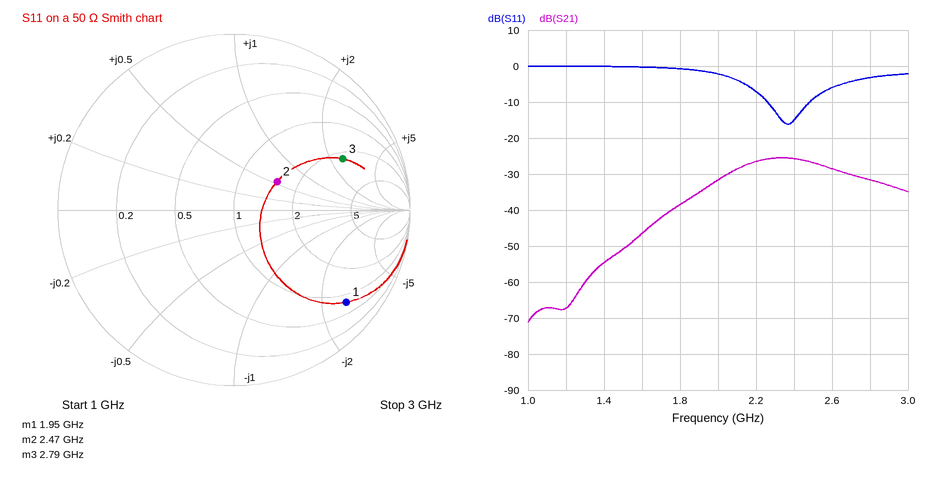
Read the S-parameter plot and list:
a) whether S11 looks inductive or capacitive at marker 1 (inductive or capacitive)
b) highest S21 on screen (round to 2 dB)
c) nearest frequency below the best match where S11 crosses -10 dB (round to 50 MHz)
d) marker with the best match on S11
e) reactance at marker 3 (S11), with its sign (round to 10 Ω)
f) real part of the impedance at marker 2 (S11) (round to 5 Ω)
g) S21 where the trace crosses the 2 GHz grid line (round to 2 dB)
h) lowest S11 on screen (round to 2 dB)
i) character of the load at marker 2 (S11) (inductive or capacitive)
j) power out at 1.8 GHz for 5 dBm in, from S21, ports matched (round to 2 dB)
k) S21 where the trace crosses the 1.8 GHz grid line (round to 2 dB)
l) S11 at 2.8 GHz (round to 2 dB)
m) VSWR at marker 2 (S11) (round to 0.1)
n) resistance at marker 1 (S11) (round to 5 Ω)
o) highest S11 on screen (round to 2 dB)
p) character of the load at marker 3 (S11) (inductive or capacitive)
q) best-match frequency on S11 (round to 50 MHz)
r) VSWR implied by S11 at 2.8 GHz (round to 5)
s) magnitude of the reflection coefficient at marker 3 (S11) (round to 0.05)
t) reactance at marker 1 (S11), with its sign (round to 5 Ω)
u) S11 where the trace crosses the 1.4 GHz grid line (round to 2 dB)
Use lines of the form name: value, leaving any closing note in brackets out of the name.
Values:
whether S11 looks inductive or capacitive at marker 1: capacitive
highest S21 on screen: -26 dB
nearest frequency below the best match where S11 crosses -10 dB: 2.25 GHz
marker with the best match on S11: marker 2
reactance at marker 3 (S11), with its sign: +130 Ω
real part of the impedance at marker 2 (S11): 75 Ω
S21 where the trace crosses the 2 GHz grid line: -32 dB
lowest S11 on screen: -16 dB
character of the load at marker 2 (S11): inductive
power out at 1.8 GHz for 5 dBm in, from S21, ports matched: -34 dBm
S21 where the trace crosses the 1.8 GHz grid line: -38 dB
S11 at 2.8 GHz: -4 dB
VSWR at marker 2 (S11): 1.8
resistance at marker 1 (S11): 40 Ω
highest S11 on screen: 0 dB
character of the load at marker 3 (S11): inductive
best-match frequency on S11: 2.35 GHz
VSWR implied by S11 at 2.8 GHz: 5
magnitude of the reflection coefficient at marker 3 (S11): 0.70
reactance at marker 1 (S11), with its sign: -130 Ω
S11 where the trace crosses the 1.4 GHz grid line: 0 dB
